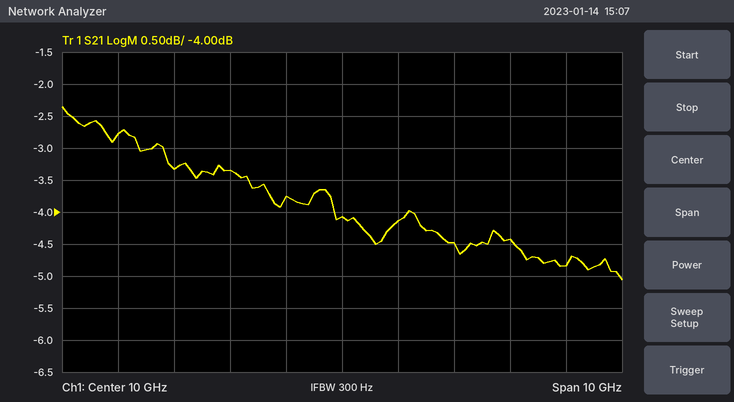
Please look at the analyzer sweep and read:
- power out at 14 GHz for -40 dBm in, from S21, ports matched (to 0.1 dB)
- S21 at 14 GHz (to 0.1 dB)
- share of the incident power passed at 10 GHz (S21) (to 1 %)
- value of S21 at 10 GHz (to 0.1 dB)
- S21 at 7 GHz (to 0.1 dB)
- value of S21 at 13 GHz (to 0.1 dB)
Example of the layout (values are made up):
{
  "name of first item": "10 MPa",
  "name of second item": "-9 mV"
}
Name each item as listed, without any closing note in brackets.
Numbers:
{
  "power out at 14 GHz for -40 dBm in, from S21, ports matched": "-44.8 dBm",
  "S21 at 14 GHz": "-4.8 dB",
  "share of the incident power passed at 10 GHz (S21)": "39 %",
  "value of S21 at 10 GHz": "-4.1 dB",
  "S21 at 7 GHz": "-3.3 dB",
  "value of S21 at 13 GHz": "-4.4 dB"
}
